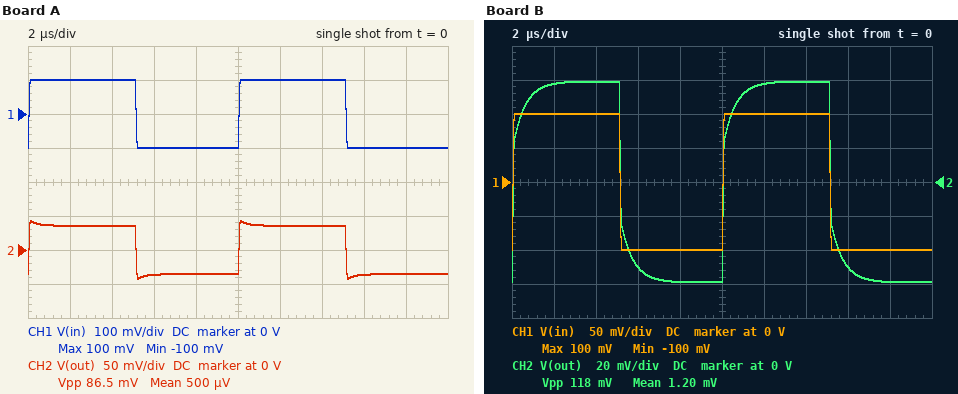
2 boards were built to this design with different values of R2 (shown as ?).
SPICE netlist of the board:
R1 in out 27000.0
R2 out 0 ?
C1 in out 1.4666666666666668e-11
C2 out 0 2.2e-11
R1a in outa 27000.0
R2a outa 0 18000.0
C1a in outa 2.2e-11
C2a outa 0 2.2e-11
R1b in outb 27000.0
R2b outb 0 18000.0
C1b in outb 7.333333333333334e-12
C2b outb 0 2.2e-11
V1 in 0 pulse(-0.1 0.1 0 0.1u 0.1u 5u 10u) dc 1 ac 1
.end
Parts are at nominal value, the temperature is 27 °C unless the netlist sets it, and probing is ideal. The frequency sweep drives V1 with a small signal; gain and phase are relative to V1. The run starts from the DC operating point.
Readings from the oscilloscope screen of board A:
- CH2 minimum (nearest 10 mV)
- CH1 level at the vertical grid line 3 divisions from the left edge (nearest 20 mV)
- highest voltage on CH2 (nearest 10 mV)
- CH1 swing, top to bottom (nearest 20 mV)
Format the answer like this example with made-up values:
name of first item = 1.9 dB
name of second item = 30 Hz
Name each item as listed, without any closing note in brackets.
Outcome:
CH2 minimum = -40 mV
CH1 level at the vertical grid line 3 divisions from the left edge = -100 mV
highest voltage on CH2 = 40 mV
CH1 swing, top to bottom = 200 mV
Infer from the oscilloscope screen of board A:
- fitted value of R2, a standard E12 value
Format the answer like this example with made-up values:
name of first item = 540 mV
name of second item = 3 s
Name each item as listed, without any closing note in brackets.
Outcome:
fitted value of R2, a standard E12 value = 15 kΩ
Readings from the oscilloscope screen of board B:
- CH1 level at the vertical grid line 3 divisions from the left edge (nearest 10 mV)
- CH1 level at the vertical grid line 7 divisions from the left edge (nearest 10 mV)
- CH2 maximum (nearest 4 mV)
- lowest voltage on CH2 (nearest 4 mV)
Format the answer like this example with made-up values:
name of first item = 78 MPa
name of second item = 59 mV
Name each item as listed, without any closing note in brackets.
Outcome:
CH1 level at the vertical grid line 3 divisions from the left edge = -100 mV
CH1 level at the vertical grid line 7 divisions from the left edge = 100 mV
CH2 maximum = 60 mV
lowest voltage on CH2 = -60 mV
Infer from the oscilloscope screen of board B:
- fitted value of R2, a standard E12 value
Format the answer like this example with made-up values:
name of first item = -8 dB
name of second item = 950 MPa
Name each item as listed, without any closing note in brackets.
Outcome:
fitted value of R2, a standard E12 value = 39 kΩ
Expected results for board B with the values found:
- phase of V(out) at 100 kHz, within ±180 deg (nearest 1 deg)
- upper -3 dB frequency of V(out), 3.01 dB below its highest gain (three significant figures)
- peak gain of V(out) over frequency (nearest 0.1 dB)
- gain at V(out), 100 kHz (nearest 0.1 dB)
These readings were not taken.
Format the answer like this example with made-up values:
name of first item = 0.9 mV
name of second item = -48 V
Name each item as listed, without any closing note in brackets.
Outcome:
phase of V(out) at 100 kHz, within ±180 deg = -6 deg
upper -3 dB frequency of V(out), 3.01 dB below its highest gain = 941 kHz
peak gain of V(out) over frequency = -4.6 dB
gain at V(out), 100 kHz = -4.9 dB
